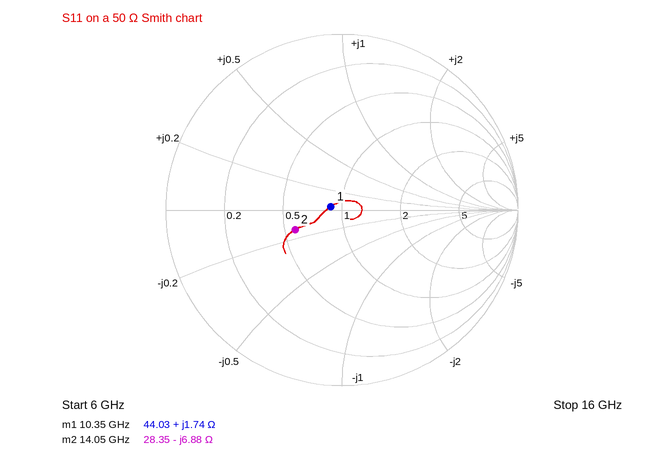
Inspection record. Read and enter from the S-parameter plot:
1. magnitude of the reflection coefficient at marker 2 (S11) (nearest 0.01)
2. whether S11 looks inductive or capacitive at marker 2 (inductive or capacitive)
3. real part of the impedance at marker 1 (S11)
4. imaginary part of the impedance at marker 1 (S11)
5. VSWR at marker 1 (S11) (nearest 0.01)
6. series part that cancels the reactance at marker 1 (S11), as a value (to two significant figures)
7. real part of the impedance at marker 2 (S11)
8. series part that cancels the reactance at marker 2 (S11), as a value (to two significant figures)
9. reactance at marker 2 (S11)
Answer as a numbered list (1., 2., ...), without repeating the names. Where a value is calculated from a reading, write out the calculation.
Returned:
1. 0.29
2. capacitive
3. 44.03 Ω
4. +1.74 Ω
5. 1.14
6. C = 1/(2π × 10.35 GHz × 1.74 Ω) ≈ 8.8 pF
7. 28.35 Ω
8. L = 6.88 Ω/(2π × 14.05 GHz) ≈ 78 pH
9. -6.88 Ω
